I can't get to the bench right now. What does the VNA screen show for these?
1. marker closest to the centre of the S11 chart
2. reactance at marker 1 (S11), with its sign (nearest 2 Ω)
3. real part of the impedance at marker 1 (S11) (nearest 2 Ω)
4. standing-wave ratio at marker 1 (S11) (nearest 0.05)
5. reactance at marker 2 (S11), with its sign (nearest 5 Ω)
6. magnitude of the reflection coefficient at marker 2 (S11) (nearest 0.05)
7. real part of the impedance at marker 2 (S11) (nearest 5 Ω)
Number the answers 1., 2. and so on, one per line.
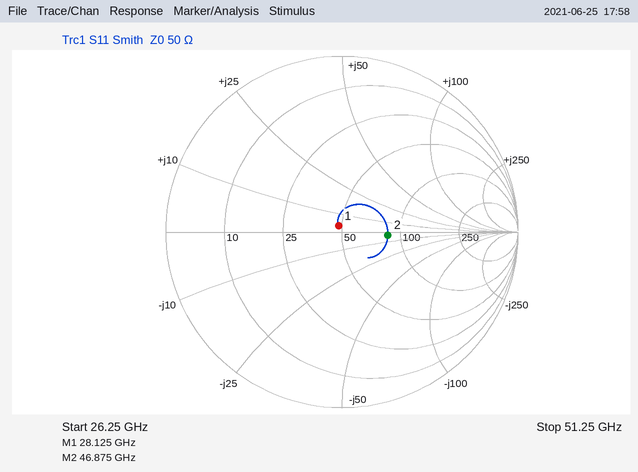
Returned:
1. marker 1
2. +4 Ω
3. 48 Ω
4. 1.10
5. -5 Ω
6. 0.25
7. 85 Ω
